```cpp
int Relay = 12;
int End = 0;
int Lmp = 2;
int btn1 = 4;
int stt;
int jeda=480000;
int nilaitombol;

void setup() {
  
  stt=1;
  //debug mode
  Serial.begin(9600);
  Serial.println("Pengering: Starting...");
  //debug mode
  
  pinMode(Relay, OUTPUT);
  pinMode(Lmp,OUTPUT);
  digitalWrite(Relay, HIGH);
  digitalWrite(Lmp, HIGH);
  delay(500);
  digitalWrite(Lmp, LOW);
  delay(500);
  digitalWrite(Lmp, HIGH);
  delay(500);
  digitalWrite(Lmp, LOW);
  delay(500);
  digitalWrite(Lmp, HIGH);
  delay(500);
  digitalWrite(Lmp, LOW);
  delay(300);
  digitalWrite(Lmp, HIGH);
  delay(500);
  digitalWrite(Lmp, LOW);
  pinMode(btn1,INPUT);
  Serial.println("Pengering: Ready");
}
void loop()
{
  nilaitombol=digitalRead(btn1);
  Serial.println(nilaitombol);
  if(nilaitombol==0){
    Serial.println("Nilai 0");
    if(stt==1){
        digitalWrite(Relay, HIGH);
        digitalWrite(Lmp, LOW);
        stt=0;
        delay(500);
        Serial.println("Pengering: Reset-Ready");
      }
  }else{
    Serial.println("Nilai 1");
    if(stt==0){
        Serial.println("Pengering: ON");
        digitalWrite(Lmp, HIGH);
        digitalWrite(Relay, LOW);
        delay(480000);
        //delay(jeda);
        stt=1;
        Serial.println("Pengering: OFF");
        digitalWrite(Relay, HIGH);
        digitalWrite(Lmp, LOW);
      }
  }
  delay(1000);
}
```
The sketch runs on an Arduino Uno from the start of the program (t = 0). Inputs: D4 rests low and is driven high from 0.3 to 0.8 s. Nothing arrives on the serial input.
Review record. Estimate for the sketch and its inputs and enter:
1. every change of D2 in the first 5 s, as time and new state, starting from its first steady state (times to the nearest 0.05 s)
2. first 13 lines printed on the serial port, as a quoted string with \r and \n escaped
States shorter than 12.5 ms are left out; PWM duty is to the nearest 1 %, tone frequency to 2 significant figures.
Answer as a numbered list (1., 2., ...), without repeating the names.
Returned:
1. 0 s high; 0.5 s low; 1 s high; 1.5 s low; 2 s high; 2.5 s low; 2.8 s high; 3.3 s low
2. "Pengering: Starting...\r\nPengering: Ready\r\n0\r\nNilai 0\r\nPengering: Reset-Ready\r\n0\r\nNilai 0\r\n0\r\nNilai 0\r\n0\r\nNilai 0\r\n0\r\nNilai 0\r\n"
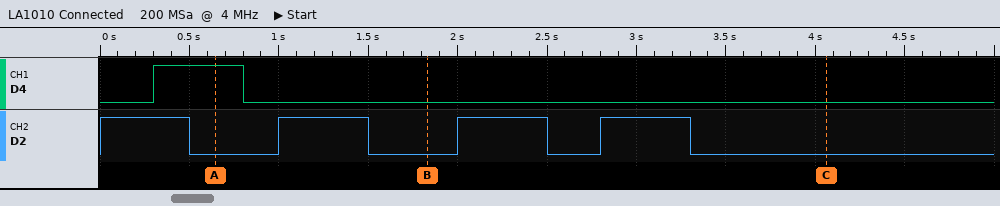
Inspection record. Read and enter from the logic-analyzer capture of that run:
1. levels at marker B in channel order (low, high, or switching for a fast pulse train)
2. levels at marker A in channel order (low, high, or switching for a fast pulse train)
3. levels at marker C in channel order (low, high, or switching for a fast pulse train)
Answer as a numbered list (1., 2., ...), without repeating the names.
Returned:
1. D4 low, D2 low
2. D4 high, D2 low
3. D4 low, D2 low
